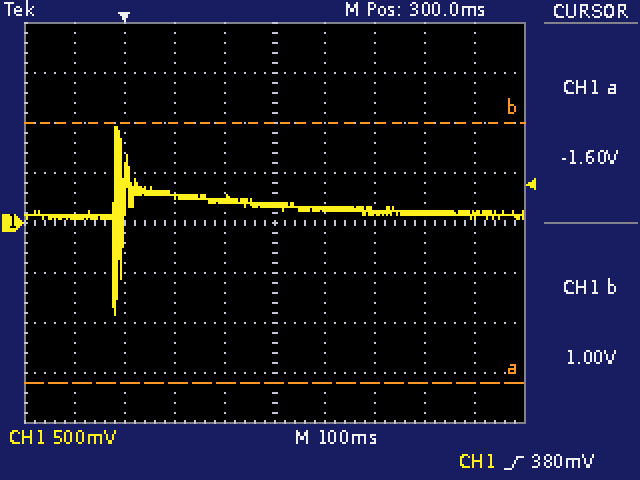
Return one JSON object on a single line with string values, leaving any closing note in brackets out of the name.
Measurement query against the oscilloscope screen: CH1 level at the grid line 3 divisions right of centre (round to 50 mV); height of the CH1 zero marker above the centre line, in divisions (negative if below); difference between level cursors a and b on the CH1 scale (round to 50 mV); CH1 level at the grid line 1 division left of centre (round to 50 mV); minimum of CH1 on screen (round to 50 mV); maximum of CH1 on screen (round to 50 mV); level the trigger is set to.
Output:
{"CH1 level at the grid line 3 divisions right of centre": "100 mV", "height of the CH1 zero marker above the centre line, in divisions": "0.0 div", "difference between level cursors a and b on the CH1 scale": "2.60 V", "CH1 level at the grid line 1 division left of centre": "250 mV", "minimum of CH1 on screen": "-900 mV", "maximum of CH1 on screen": "950 mV", "level the trigger is set to": "380 mV"}
